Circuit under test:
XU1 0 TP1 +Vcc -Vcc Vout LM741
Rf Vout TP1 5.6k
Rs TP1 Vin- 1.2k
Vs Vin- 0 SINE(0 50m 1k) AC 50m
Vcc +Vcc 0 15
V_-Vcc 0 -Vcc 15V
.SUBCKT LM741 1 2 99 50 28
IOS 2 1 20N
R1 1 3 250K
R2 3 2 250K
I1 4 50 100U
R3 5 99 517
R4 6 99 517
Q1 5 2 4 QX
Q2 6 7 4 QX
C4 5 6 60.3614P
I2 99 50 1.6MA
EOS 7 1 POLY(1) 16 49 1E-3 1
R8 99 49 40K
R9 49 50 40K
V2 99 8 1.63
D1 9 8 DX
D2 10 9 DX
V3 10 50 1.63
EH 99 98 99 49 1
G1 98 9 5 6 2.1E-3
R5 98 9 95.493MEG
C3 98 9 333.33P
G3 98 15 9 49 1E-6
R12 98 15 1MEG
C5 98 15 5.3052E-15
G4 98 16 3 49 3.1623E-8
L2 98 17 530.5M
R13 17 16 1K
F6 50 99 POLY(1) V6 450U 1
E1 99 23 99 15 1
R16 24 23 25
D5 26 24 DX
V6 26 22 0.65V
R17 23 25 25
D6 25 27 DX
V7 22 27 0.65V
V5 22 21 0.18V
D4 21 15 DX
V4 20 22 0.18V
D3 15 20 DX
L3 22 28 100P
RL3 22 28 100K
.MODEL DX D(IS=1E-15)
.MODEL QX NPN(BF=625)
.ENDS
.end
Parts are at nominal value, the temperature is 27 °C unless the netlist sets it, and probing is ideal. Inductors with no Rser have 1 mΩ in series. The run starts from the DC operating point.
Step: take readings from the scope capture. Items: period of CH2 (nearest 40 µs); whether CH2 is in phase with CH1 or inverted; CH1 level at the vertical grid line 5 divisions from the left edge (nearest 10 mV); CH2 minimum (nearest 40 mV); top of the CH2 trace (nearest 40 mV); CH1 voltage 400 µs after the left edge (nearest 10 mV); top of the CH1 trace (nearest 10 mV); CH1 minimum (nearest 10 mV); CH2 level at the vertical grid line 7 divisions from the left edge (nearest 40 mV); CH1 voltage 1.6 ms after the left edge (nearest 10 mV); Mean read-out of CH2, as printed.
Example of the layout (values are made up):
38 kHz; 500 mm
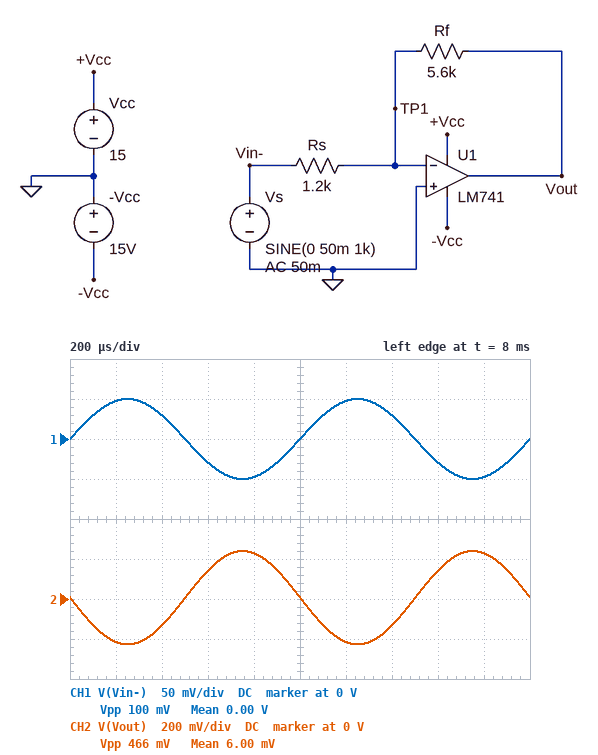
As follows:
1.00 ms; inverted; 0 V; -240 mV; 240 mV; 30 mV; 50 mV; -50 mV; -120 mV; -30 mV; 6.00 mV
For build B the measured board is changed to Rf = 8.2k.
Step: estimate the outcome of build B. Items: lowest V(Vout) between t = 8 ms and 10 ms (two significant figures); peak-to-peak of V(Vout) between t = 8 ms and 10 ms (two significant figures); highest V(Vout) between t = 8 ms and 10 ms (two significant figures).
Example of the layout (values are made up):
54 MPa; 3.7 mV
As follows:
-330 mV; 680 mV; 350 mV
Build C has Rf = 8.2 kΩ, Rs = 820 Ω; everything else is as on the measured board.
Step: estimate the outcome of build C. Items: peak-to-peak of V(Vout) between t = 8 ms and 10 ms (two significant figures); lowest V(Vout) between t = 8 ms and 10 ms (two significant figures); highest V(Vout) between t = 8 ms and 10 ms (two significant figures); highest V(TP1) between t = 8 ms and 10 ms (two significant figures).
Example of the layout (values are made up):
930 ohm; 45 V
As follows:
1.0 V; -490 mV; 510 mV; 1.5 mV
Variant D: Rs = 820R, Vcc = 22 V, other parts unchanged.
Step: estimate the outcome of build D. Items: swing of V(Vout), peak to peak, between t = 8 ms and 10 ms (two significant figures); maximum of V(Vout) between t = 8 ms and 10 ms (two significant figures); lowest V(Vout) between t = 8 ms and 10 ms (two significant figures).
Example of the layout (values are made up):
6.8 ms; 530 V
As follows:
680 mV; 350 mV; -330 mV
